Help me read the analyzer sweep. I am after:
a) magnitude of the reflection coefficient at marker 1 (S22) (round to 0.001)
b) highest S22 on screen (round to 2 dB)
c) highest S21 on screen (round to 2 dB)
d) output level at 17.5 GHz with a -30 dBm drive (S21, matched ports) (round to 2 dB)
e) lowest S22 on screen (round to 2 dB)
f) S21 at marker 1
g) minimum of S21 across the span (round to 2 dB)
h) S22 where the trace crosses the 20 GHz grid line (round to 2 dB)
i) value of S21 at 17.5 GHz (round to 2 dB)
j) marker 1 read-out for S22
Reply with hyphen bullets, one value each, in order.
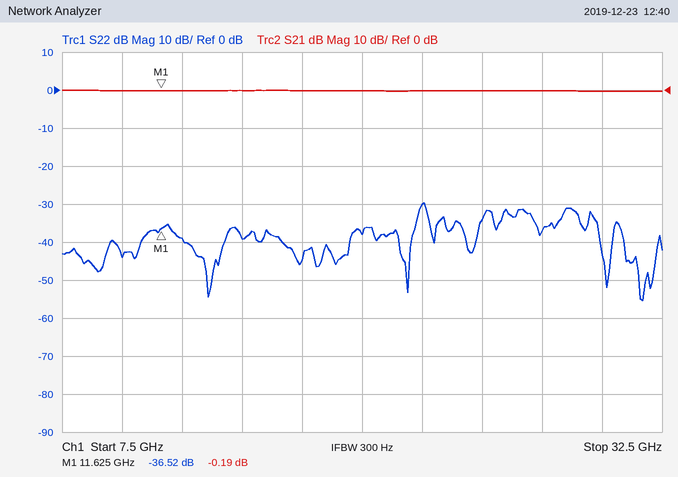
- 0.015
- -30 dB
- 0 dB
- -30 dBm
- -56 dB
- -0.19 dB
- 0 dB
- -38 dB
- 0 dB
- -36.52 dB
